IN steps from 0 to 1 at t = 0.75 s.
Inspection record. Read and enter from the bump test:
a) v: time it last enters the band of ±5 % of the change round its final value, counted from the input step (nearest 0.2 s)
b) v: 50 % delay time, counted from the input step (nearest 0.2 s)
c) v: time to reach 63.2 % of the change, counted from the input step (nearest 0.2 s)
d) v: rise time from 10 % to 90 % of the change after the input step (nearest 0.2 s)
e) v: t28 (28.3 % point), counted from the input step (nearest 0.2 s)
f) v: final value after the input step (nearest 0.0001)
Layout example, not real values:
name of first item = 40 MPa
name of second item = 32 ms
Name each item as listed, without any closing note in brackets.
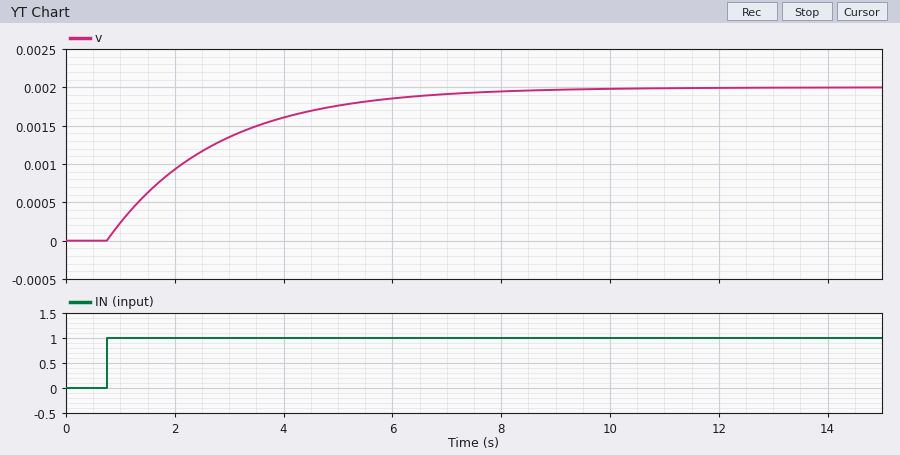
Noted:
v: time it last enters the band of ±5 % of the change round its final value, counted from the input step = 6.0 s
v: 50 % delay time, counted from the input step = 1.4 s
v: time to reach 63.2 % of the change, counted from the input step = 2.0 s
v: rise time from 10 % to 90 % of the change after the input step = 4.4 s
v: t28 (28.3 % point), counted from the input step = 0.6 s
v: final value after the input step = 0.0020
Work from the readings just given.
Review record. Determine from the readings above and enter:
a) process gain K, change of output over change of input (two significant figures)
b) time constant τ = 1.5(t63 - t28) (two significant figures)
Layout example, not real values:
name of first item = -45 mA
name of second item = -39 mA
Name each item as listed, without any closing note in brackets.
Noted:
process gain K, change of output over change of input = 0.0020
time constant τ = 1.5(t63 - t28) = 2.1 s
